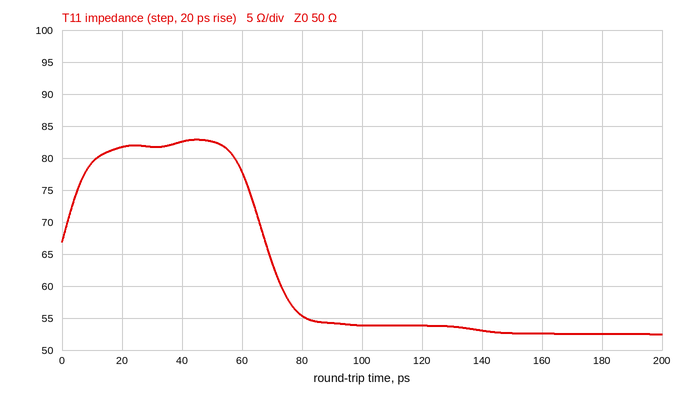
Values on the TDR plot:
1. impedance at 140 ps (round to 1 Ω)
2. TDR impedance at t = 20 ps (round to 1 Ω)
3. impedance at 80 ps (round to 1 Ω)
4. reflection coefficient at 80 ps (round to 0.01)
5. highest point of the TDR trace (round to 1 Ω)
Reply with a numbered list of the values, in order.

1. 53 Ω
2. 82 Ω
3. 55 Ω
4. +0.05
5. 83 Ω
